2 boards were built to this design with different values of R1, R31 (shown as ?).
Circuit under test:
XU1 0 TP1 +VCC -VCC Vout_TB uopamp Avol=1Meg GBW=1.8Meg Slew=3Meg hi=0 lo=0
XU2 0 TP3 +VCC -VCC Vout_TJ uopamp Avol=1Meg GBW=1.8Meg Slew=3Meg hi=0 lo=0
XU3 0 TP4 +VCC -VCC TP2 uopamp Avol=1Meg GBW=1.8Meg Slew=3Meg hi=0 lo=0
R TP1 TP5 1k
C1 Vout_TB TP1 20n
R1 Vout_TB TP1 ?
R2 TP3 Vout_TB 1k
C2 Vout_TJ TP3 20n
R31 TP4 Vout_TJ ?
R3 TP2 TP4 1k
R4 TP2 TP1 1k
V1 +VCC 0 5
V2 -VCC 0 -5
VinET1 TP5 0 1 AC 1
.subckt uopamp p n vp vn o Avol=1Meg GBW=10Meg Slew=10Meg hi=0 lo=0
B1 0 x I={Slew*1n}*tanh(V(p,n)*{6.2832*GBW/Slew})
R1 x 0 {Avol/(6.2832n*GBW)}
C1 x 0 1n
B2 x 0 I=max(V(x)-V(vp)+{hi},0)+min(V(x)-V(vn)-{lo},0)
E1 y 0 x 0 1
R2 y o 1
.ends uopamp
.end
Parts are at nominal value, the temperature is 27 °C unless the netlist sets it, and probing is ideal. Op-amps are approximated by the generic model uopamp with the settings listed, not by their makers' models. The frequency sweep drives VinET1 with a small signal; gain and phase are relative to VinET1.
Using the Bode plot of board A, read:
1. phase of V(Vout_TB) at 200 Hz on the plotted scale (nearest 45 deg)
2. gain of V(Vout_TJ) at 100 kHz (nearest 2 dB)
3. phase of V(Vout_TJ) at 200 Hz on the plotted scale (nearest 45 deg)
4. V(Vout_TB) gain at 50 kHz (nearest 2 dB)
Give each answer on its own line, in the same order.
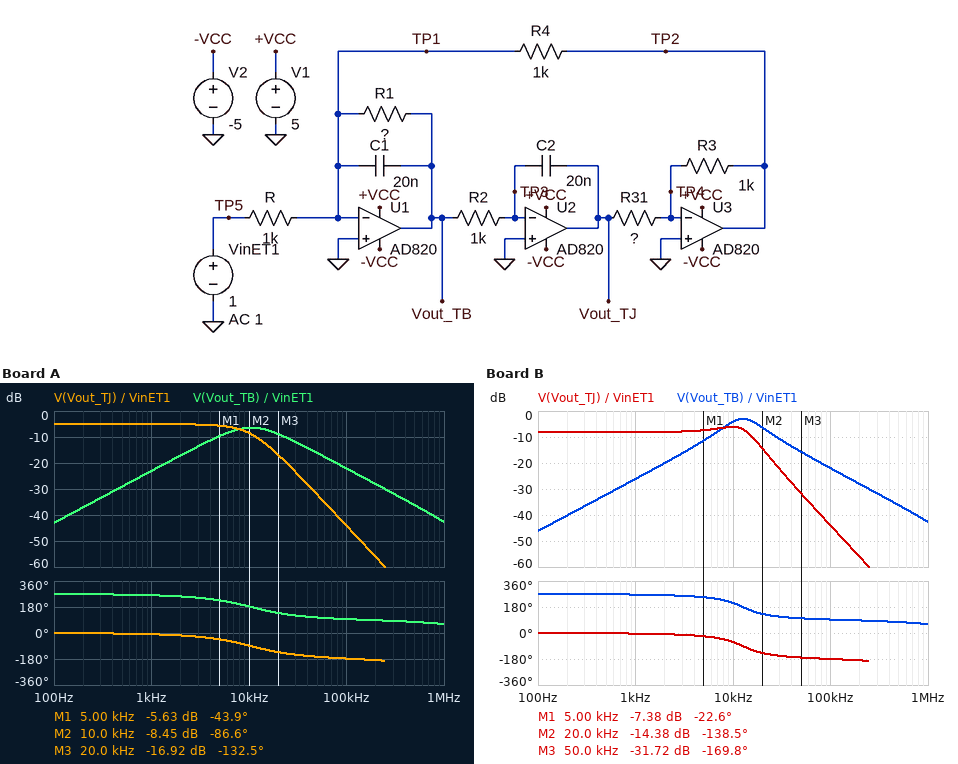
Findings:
270 deg
-44 dB
0 deg
-16 dB
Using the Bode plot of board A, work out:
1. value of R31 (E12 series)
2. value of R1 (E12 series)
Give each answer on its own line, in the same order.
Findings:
560 Ω
470 Ω
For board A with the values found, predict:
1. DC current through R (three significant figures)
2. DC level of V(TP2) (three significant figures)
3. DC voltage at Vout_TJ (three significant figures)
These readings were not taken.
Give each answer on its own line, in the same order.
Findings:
1.00 mA
-1.00 V
560 mV
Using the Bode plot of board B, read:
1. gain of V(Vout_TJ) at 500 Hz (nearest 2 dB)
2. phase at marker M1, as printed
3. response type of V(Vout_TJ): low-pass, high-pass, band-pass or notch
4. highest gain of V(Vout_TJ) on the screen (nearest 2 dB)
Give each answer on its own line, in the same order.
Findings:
-8 dB
-22.6 deg
low-pass
-6 dB
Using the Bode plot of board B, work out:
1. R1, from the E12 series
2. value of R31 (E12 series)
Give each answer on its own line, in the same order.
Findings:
680 Ω
390 Ω
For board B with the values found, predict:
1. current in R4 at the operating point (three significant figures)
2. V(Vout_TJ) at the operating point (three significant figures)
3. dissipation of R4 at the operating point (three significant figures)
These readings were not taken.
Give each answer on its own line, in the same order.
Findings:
1.00 mA
390 mV
1.00 mW
